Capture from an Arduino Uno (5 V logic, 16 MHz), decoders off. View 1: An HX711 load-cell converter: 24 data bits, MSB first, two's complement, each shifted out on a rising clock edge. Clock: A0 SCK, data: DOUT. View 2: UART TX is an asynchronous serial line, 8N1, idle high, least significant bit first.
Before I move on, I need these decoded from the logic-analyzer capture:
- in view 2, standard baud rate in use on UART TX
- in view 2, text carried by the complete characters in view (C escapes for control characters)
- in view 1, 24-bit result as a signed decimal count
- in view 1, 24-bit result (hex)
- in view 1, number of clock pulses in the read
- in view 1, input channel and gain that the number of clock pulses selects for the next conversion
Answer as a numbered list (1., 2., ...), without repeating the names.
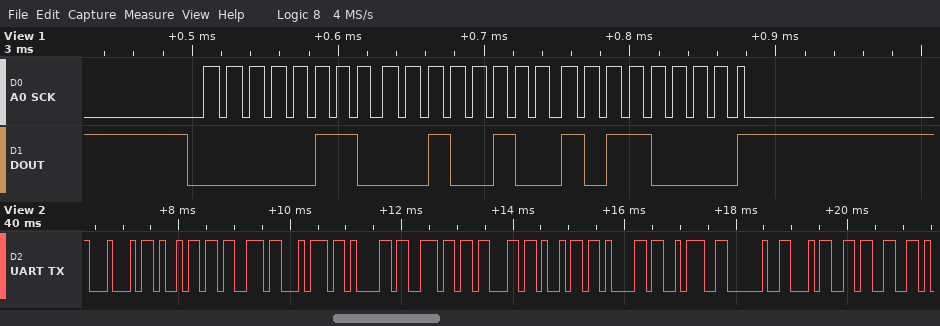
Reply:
1. 9600 baud
2. "Distancia: 43"
3. 402608
4. 0x0624B0
5. 25
6. channel A, gain 128
